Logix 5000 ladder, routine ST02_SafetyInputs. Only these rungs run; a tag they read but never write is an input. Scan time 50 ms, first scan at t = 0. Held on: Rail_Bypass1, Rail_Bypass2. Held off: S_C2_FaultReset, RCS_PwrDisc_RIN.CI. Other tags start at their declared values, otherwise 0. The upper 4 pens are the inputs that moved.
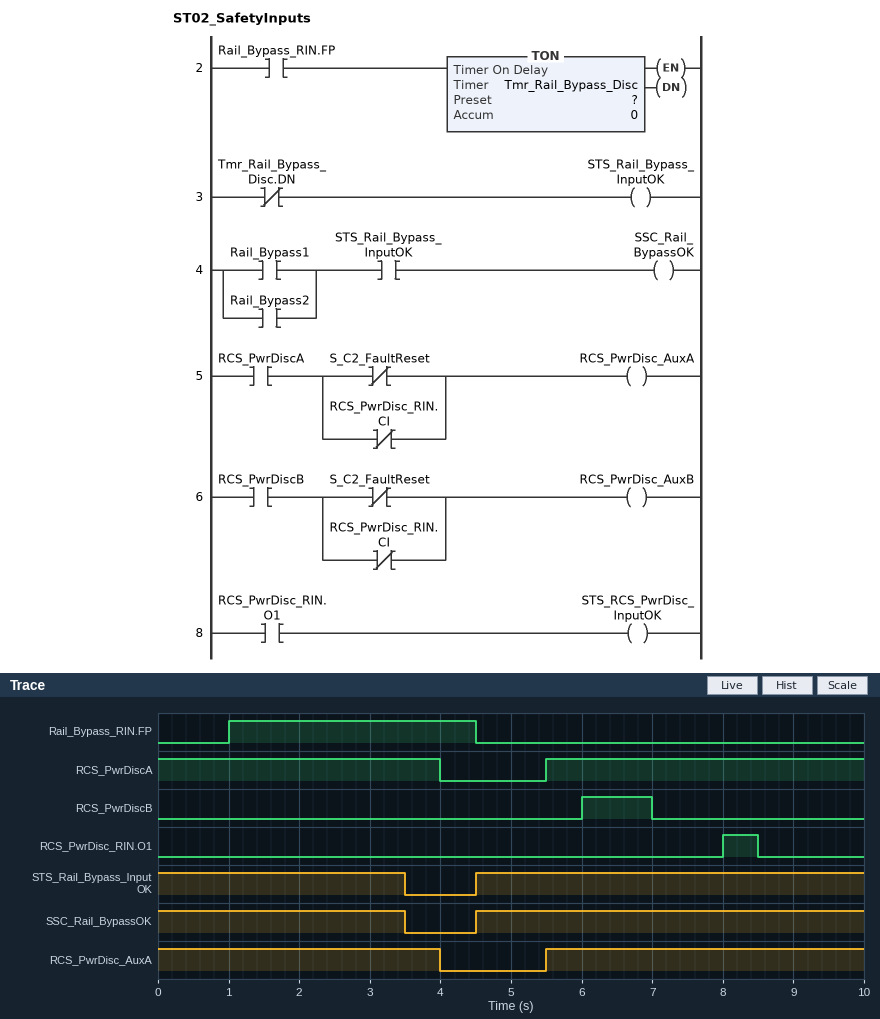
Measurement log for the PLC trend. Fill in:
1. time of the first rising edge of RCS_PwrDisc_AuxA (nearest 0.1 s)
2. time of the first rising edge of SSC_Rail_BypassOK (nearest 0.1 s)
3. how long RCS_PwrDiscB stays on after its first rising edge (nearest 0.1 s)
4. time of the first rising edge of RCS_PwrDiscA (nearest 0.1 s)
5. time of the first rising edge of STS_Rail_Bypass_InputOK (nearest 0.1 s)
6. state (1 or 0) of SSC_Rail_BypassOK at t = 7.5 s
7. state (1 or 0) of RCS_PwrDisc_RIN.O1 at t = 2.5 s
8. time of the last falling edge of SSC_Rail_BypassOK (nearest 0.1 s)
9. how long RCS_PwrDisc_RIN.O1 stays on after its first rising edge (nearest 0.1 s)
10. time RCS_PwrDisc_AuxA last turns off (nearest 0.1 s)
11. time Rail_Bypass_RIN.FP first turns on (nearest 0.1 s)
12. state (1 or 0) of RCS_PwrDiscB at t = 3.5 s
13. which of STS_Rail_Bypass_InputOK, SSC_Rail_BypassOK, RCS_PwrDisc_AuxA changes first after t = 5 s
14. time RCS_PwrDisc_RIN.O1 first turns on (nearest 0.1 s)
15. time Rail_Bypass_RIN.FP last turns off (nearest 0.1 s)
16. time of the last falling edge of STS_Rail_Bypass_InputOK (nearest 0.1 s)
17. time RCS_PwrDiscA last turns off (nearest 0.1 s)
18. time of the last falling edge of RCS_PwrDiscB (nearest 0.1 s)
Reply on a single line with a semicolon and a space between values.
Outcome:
5.5 s; 4.5 s; 1.0 s; 5.5 s; 4.5 s; 1; 0; 3.5 s; 0.5 s; 4.0 s; 1.0 s; 0; RCS_PwrDisc_AuxA; 8.0 s; 4.5 s; 3.5 s; 4.0 s; 7.0 s
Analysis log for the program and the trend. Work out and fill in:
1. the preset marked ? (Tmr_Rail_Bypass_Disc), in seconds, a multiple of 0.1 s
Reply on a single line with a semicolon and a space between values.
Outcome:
2.5 s
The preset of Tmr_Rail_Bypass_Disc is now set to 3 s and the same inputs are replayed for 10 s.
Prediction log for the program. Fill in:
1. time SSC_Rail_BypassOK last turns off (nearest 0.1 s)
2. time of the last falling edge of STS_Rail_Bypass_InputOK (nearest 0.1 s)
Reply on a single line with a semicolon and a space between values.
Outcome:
4.0 s; 4.0 s
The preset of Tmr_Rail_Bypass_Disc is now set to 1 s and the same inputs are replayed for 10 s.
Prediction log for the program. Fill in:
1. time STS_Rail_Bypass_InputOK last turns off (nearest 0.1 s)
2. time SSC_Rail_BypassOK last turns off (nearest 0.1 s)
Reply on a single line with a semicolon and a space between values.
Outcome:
2.0 s; 2.0 s
